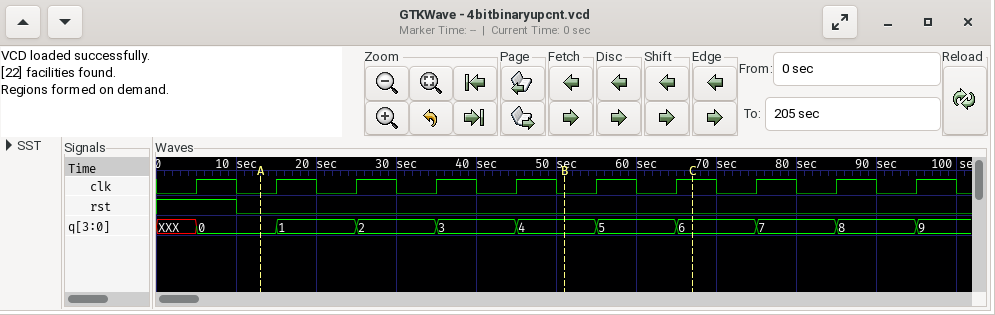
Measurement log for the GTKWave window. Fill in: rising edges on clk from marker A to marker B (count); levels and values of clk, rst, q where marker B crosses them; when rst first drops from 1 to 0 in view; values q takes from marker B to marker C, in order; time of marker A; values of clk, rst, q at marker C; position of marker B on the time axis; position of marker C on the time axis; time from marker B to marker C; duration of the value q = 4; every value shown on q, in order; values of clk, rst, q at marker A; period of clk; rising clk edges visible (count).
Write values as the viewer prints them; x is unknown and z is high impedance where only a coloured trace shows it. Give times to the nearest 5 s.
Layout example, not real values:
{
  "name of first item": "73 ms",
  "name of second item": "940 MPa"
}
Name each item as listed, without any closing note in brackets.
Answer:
{
  "rising edges on clk from marker A to marker B": "4",
  "levels and values of clk, rst, q where marker B crosses them": "clk=0, rst=0, q=4",
  "when rst first drops from 1 to 0 in view": "10 s",
  "values q takes from marker B to marker C, in order": "4, 5, 6",
  "time of marker A": "15 s",
  "values of clk, rst, q at marker C": "clk=1, rst=0, q=6",
  "position of marker B on the time axis": "50 s",
  "position of marker C on the time axis": "65 s",
  "time from marker B to marker C": "15 s",
  "duration of the value q = 4": "10 s",
  "every value shown on q, in order": "XXX, 0, 1, 2, 3, 4, 5, 6, 7, 8, 9",
  "values of clk, rst, q at marker A": "clk=0, rst=0, q=0",
  "period of clk": "10 s",
  "rising clk edges visible": "10"
}
